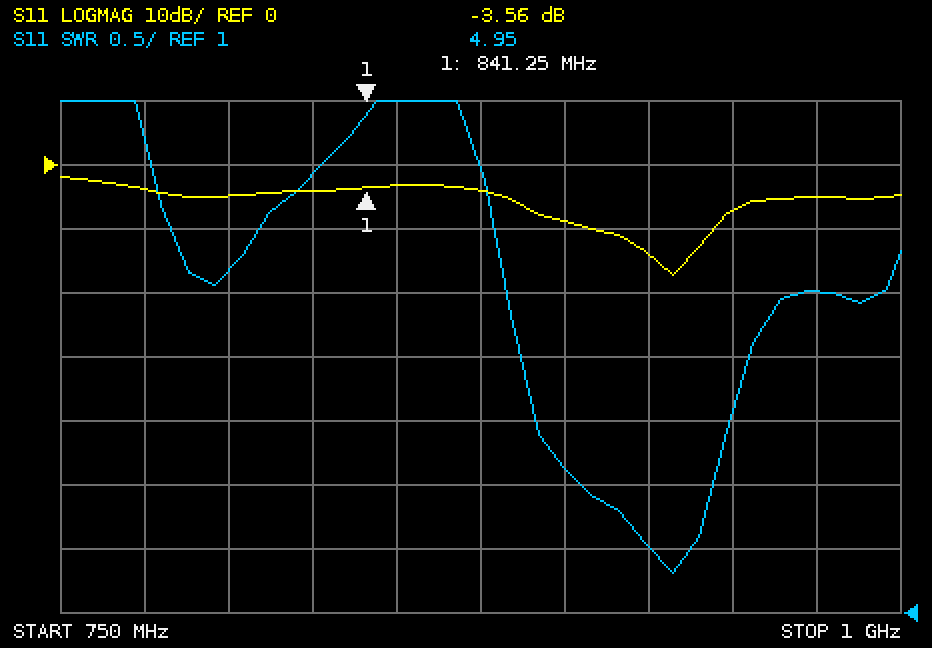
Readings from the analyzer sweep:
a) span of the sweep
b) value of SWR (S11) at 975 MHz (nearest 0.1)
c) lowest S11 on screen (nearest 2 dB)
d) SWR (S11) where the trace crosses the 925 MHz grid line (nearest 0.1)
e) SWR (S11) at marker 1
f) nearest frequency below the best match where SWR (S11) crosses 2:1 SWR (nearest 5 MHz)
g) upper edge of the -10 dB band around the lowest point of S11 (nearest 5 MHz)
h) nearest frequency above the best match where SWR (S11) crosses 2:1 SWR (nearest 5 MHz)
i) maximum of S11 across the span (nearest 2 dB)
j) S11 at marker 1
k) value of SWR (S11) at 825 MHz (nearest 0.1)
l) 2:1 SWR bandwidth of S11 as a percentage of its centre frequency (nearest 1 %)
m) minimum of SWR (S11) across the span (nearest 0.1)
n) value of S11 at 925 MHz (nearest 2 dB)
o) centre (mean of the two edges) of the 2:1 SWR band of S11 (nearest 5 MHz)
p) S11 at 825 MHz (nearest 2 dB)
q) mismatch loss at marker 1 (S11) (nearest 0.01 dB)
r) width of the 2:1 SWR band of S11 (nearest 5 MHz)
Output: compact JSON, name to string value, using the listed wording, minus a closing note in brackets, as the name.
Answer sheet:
{"span of the sweep": "250 MHz", "value of SWR (S11) at 975 MHz": "3.5", "lowest S11 on screen": "-18 dB", "SWR (S11) where the trace crosses the 925 MHz grid line": "1.5", "SWR (S11) at marker 1": "4.95", "nearest frequency below the best match where SWR (S11) crosses 2:1 SWR": "905 MHz", "upper edge of the -10 dB band around the lowest point of S11": "945 MHz", "nearest frequency above the best match where SWR (S11) crosses 2:1 SWR": "945 MHz", "maximum of S11 across the span": "-2 dB", "S11 at marker 1": "-3.56 dB", "value of SWR (S11) at 825 MHz": "4.4", "2:1 SWR bandwidth of S11 as a percentage of its centre frequency": "4 %", "minimum of SWR (S11) across the span": "1.3", "value of S11 at 925 MHz": "-14 dB", "centre (mean of the two edges) of the 2:1 SWR band of S11": "925 MHz", "S11 at 825 MHz": "-4 dB", "mismatch loss at marker 1 (S11)": "2.52 dB", "width of the 2:1 SWR band of S11": "40 MHz"}
